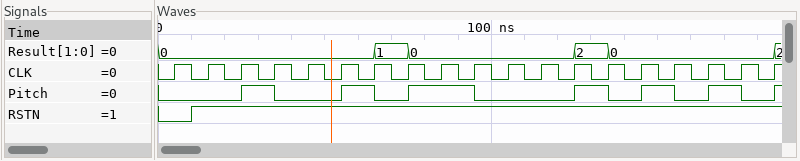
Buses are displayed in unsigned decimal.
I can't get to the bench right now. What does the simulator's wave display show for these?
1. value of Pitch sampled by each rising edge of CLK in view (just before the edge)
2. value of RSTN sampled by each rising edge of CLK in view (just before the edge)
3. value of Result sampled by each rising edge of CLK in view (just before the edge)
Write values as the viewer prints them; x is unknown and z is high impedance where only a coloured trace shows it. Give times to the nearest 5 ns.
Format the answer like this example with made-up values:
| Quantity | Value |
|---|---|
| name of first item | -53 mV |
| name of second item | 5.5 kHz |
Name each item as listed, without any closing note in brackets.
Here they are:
| Quantity | Value |
|---|---|
| value of Pitch sampled by each rising edge of CLK in view | 0 0 0 1 0 0 1 0 1 1 0 0 0 1 0 1 0 1 0 |
| value of RSTN sampled by each rising edge of CLK in view | 0 1 1 1 1 1 1 1 1 1 1 1 1 1 1 1 1 1 1 |
| value of Result sampled by each rising edge of CLK in view | 0, 0, 0, 0, 0, 0, 0, 1, 0, 0, 0, 0, 0, 2, 0, 0, 0, 0, 0 |
